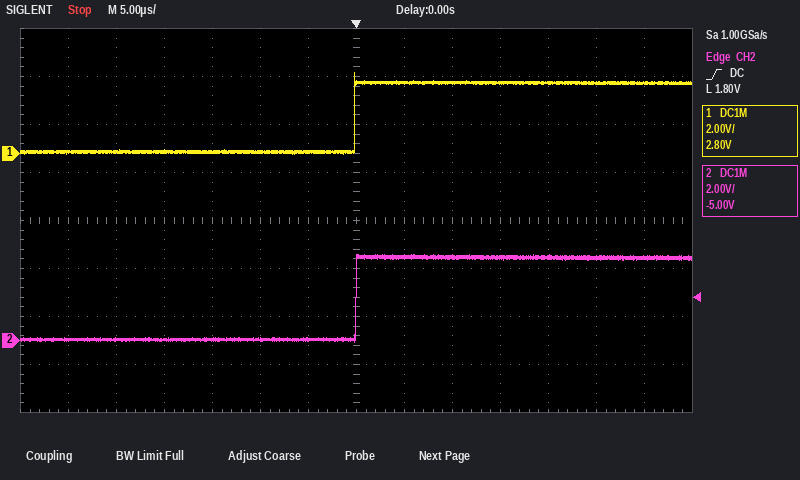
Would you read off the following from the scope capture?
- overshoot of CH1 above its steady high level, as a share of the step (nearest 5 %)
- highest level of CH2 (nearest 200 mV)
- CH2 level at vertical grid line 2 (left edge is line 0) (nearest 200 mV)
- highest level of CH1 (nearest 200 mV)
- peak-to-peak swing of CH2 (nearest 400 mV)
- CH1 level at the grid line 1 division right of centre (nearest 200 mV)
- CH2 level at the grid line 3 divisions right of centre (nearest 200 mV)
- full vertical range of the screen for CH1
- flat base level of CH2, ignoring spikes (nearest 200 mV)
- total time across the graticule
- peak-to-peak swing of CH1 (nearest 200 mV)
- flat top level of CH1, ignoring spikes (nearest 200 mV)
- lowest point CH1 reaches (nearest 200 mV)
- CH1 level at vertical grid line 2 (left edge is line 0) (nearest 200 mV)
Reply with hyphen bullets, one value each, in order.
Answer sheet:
- 15 %
- 3.6 V
- 0.0 V
- 3.4 V
- 3.6 V
- 3.0 V
- 3.4 V
- 16 V
- 0.0 V
- 70 µs
- 3.4 V
- 3.0 V
- 0.0 V
- 0.0 V
